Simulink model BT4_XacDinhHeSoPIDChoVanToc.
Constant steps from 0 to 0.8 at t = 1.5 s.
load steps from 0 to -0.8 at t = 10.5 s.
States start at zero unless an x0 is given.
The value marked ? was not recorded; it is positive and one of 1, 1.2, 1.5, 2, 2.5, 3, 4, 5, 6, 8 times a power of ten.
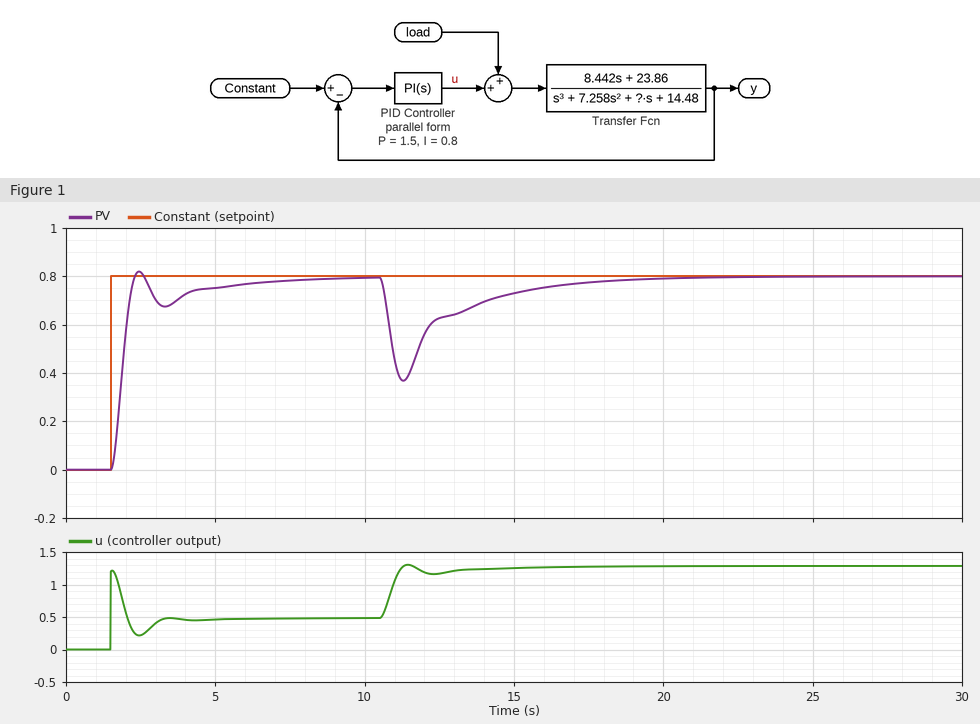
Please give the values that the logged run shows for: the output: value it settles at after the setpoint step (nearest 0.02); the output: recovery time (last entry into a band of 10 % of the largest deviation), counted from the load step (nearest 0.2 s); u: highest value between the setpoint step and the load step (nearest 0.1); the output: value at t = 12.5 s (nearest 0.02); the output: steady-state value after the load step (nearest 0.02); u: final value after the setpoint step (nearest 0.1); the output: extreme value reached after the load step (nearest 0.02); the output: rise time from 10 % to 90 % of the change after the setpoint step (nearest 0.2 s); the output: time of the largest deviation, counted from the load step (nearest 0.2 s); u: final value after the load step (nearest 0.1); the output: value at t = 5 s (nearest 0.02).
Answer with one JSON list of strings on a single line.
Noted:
["0.80", "5.8 s", "1.2", "0.62", "0.80", "0.5", "0.36", "0.6 s", "0.8 s", "1.3", "0.76"]
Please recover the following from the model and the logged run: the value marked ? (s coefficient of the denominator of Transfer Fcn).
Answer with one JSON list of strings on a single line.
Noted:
["15"]
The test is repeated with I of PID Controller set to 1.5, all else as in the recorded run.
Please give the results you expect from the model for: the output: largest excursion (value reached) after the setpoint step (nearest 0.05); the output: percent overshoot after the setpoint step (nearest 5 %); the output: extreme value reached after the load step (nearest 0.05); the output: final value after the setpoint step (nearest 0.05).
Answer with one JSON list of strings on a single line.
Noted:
["0.90", "15 %", "0.40", "0.80"]
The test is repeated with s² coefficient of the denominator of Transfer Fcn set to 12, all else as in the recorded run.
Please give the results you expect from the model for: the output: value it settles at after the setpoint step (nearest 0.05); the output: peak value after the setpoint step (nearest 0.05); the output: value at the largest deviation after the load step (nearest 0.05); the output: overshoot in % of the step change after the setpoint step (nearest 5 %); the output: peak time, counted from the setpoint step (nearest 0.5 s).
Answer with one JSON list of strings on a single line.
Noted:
["0.80", "0.85", "0.40", "10 %", "1.5 s"]
